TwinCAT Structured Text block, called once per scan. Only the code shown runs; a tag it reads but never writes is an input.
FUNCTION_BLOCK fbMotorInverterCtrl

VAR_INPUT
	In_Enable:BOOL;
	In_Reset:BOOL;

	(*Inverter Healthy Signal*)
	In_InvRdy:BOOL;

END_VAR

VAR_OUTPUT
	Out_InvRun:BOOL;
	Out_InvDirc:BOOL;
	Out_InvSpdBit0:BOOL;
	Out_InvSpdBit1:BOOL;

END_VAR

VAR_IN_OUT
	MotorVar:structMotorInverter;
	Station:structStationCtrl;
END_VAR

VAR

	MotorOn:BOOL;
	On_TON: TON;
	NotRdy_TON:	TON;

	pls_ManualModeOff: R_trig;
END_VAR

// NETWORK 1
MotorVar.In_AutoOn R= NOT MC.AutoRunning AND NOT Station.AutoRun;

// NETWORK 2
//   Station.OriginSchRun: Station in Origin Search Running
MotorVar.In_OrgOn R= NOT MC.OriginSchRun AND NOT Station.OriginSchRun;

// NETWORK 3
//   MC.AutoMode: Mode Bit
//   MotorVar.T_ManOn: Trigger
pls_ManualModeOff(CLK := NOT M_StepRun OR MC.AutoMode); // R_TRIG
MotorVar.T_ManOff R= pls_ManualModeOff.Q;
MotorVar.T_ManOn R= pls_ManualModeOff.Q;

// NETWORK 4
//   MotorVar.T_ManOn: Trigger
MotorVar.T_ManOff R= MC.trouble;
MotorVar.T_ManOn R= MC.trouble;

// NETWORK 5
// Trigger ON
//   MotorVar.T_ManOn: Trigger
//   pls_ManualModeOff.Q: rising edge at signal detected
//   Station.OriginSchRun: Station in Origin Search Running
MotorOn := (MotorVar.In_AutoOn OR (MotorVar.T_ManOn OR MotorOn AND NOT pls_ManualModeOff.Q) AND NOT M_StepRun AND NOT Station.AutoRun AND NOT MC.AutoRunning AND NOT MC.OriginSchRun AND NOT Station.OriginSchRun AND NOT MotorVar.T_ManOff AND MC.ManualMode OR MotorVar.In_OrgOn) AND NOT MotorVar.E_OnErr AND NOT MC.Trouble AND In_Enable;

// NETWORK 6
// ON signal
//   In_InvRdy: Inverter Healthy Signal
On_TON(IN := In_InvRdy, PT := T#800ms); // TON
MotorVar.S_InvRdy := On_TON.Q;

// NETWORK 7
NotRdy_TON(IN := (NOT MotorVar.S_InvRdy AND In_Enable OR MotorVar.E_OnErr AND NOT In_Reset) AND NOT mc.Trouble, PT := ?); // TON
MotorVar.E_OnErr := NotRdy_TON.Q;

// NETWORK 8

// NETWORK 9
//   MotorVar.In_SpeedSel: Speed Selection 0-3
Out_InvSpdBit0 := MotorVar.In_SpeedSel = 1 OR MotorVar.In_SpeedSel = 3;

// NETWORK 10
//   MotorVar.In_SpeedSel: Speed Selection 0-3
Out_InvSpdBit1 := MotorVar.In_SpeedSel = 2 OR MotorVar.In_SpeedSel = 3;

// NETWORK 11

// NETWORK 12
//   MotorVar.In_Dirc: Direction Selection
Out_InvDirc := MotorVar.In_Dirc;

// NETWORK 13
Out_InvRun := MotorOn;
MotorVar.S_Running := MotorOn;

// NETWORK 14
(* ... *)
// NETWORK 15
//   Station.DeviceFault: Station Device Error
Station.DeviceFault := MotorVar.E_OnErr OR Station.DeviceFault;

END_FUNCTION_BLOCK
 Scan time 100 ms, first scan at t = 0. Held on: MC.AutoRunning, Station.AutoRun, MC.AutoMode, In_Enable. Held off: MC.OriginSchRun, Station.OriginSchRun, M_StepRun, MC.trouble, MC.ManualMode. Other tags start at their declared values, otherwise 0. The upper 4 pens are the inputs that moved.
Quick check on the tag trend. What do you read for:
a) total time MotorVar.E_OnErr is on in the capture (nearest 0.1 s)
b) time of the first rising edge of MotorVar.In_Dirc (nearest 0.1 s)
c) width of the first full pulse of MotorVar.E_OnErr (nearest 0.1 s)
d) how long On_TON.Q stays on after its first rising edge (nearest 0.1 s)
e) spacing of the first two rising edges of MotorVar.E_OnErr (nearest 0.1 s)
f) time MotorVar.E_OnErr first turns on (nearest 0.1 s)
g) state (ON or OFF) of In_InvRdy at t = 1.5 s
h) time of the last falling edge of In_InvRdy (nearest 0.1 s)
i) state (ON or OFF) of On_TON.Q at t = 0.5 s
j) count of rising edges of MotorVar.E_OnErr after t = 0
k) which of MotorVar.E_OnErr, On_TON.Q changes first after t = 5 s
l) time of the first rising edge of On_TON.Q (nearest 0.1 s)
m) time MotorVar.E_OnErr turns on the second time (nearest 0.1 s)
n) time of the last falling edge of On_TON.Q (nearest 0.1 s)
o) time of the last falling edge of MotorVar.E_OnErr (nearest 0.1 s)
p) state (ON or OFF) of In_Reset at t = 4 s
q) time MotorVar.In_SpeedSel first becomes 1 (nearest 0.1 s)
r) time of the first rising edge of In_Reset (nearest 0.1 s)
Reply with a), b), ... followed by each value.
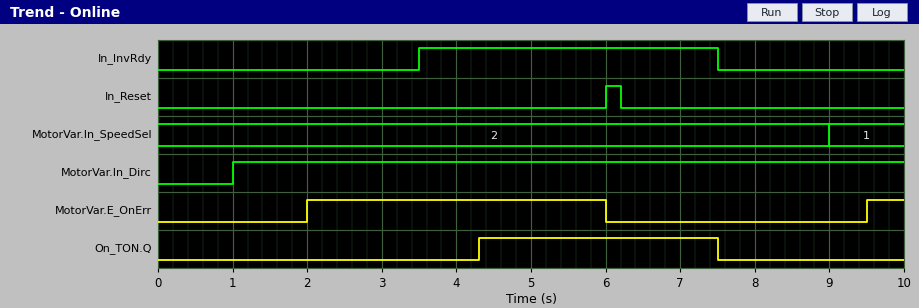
a) 4.5 s
b) 1.0 s
c) 4.0 s
d) 3.2 s
e) 7.5 s
f) 2.0 s
g) OFF
h) 7.5 s
i) OFF
j) 2
k) MotorVar.E_OnErr
l) 4.3 s
m) 9.5 s
n) 7.5 s
o) 6.0 s
p) OFF
q) 9.0 s
r) 6.0 s
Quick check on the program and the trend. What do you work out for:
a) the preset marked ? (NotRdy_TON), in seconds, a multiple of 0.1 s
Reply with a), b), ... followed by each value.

a) 2.0 s
